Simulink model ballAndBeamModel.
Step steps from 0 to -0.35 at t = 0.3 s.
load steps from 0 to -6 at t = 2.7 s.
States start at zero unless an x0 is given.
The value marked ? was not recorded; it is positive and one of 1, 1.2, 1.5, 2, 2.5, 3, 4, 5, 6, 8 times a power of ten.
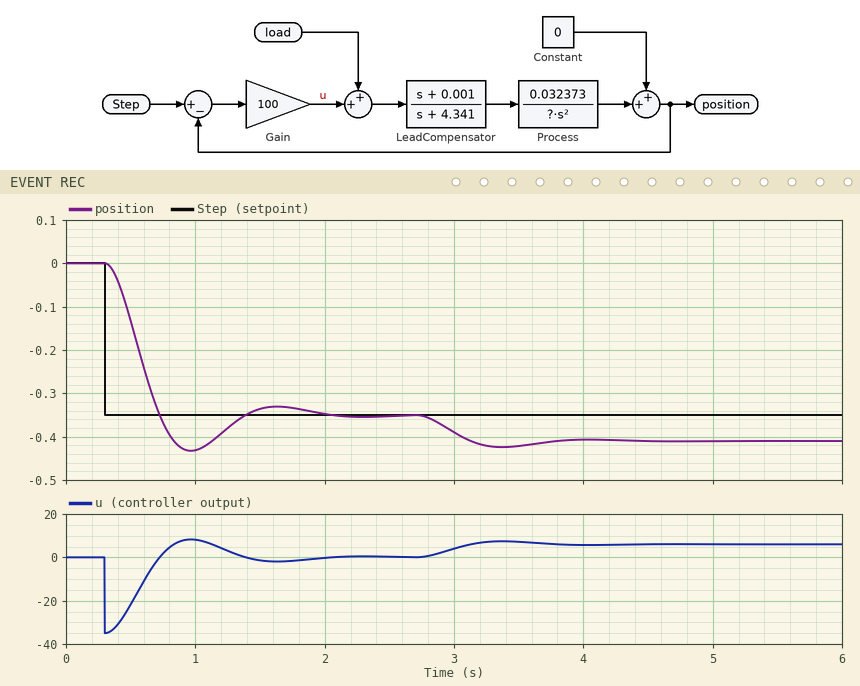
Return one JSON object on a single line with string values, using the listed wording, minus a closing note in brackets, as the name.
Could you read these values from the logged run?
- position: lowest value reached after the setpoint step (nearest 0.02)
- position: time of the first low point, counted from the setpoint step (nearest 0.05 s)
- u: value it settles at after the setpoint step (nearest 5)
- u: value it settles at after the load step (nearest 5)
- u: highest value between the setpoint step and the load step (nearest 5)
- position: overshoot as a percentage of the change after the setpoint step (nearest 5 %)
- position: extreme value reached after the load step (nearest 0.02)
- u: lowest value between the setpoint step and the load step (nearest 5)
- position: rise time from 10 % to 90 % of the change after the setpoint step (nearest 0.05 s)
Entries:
{"position: lowest value reached after the setpoint step": "-0.44", "position: time of the first low point, counted from the setpoint step": "0.65 s", "u: value it settles at after the setpoint step": "0", "u: value it settles at after the load step": "5", "u: highest value between the setpoint step and the load step": "10", "position: overshoot as a percentage of the change after the setpoint step": "25 %", "position: extreme value reached after the load step": "-0.42", "u: lowest value between the setpoint step and the load step": "-35", "position: rise time from 10 % to 90 % of the change after the setpoint step": "0.30 s"}
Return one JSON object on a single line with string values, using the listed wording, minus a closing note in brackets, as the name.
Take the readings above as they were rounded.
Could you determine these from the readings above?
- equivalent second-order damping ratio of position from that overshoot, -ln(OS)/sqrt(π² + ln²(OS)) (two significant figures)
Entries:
{"equivalent second-order damping ratio of position from that overshoot, -ln(OS)/sqrt(π² + ln²(OS))": "0.40"}
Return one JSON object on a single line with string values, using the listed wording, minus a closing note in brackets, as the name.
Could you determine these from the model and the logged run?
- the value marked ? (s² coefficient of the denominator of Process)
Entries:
{"the value marked ?": "0.12"}
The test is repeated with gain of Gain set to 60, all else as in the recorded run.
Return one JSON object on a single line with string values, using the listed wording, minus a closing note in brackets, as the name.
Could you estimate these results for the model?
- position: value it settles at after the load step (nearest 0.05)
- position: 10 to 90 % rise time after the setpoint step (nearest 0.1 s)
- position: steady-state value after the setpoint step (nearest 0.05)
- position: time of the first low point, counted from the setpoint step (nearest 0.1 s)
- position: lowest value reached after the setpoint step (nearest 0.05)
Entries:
{"position: value it settles at after the load step": "-0.45", "position: 10 to 90 % rise time after the setpoint step": "0.4 s", "position: steady-state value after the setpoint step": "-0.35", "position: time of the first low point, counted from the setpoint step": "0.9 s", "position: lowest value reached after the setpoint step": "-0.40"}
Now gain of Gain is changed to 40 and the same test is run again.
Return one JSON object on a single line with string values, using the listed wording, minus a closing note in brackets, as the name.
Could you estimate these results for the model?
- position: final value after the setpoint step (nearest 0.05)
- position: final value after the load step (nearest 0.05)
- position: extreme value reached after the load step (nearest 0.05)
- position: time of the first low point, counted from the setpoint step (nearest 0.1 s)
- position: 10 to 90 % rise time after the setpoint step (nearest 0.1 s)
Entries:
{"position: final value after the setpoint step": "-0.35", "position: final value after the load step": "-0.50", "position: extreme value reached after the load step": "-0.50", "position: time of the first low point, counted from the setpoint step": "1.3 s", "position: 10 to 90 % rise time after the setpoint step": "0.6 s"}
